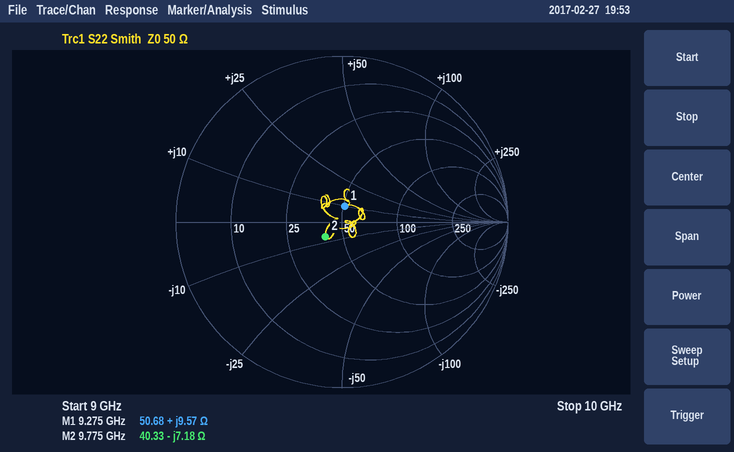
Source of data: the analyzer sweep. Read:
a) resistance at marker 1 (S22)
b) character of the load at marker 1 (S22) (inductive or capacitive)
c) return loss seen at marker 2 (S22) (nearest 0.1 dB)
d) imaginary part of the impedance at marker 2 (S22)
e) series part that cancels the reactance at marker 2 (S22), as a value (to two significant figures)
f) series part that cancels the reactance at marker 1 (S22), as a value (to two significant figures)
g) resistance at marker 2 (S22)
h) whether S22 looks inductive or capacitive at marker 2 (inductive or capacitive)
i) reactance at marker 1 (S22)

50.68 Ω
inductive
17.5 dB
-7.18 Ω
120 pH
1.8 pF
40.33 Ω
capacitive
+9.57 Ω
